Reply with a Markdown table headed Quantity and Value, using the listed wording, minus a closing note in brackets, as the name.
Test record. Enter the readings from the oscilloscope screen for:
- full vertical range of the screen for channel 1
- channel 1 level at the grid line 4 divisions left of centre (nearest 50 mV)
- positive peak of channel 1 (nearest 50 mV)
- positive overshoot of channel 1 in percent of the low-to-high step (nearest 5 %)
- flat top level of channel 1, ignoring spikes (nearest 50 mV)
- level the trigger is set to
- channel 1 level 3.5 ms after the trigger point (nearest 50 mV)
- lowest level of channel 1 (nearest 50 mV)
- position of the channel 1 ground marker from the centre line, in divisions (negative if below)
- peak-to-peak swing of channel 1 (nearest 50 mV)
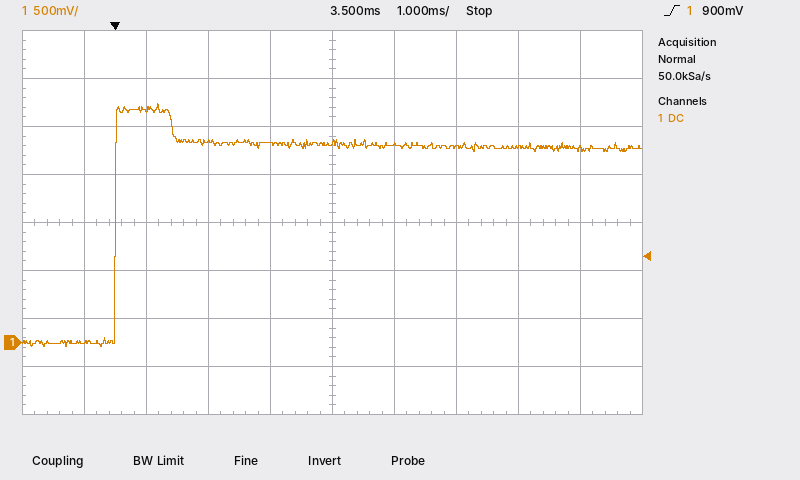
| Quantity | Value |
|---|---|
| full vertical range of the screen for channel 1 | 4 V |
| channel 1 level at the grid line 4 divisions left of centre | 0 mV |
| positive peak of channel 1 | 2.50 V |
| positive overshoot of channel 1 in percent of the low-to-high step | 20 % |
| flat top level of channel 1, ignoring spikes | 2.05 V |
| level the trigger is set to | 900 mV |
| channel 1 level 3.5 ms after the trigger point | 2.10 V |
| lowest level of channel 1 | -50 mV |
| position of the channel 1 ground marker from the centre line, in divisions | -2.5 div |
| peak-to-peak swing of channel 1 | 2.55 V |
